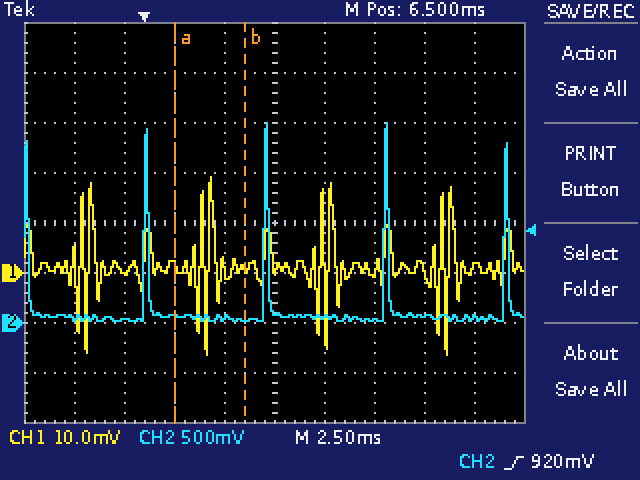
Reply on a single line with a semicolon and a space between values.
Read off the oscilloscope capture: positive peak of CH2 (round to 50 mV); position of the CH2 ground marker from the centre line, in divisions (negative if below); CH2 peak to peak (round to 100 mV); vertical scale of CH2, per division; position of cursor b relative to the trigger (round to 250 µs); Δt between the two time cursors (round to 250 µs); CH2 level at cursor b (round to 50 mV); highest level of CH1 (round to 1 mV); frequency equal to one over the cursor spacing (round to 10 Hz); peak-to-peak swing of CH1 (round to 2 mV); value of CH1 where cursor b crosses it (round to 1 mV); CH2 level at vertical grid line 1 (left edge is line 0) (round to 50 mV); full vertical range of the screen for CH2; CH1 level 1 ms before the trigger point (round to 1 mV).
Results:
2.00 V; -2.0 div; 2.00 V; 500 mV; +5.00 ms; 3.50 ms; 50 mV; 19 mV; 290 Hz; 36 mV; 1 mV; 50 mV; 4 V; 0 mV
